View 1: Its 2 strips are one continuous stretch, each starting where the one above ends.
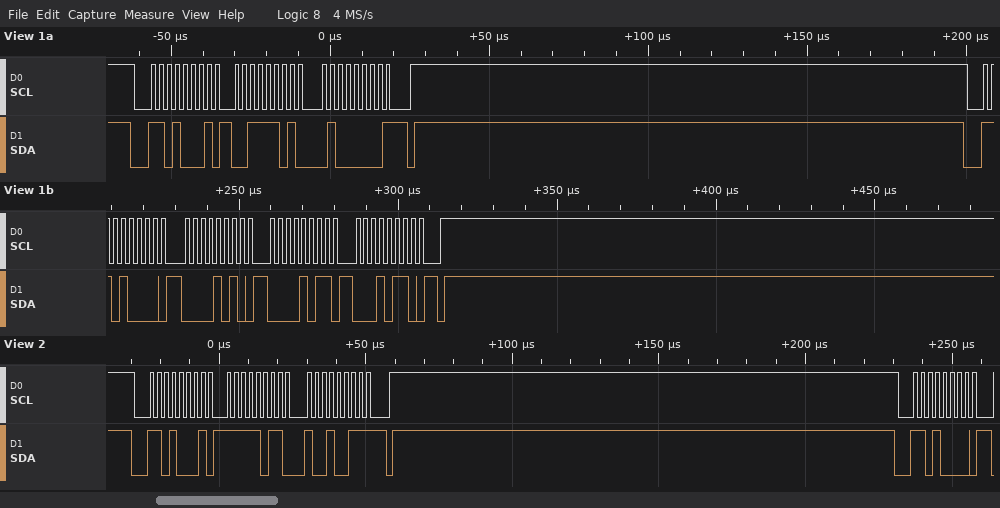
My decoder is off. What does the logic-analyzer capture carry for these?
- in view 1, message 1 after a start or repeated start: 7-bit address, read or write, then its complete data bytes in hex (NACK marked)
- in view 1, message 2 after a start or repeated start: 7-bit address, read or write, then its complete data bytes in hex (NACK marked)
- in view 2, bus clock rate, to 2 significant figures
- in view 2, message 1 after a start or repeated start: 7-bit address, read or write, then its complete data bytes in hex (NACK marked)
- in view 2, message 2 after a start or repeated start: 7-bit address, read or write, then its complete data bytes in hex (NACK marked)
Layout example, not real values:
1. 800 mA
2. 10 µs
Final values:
1. 0x68 read: 3D 40 NACK
2. 0x68 write: 0A 0B 16
3. 400 kHz
4. 0x68 read: FB 93 NACK
5. 0x68 write
